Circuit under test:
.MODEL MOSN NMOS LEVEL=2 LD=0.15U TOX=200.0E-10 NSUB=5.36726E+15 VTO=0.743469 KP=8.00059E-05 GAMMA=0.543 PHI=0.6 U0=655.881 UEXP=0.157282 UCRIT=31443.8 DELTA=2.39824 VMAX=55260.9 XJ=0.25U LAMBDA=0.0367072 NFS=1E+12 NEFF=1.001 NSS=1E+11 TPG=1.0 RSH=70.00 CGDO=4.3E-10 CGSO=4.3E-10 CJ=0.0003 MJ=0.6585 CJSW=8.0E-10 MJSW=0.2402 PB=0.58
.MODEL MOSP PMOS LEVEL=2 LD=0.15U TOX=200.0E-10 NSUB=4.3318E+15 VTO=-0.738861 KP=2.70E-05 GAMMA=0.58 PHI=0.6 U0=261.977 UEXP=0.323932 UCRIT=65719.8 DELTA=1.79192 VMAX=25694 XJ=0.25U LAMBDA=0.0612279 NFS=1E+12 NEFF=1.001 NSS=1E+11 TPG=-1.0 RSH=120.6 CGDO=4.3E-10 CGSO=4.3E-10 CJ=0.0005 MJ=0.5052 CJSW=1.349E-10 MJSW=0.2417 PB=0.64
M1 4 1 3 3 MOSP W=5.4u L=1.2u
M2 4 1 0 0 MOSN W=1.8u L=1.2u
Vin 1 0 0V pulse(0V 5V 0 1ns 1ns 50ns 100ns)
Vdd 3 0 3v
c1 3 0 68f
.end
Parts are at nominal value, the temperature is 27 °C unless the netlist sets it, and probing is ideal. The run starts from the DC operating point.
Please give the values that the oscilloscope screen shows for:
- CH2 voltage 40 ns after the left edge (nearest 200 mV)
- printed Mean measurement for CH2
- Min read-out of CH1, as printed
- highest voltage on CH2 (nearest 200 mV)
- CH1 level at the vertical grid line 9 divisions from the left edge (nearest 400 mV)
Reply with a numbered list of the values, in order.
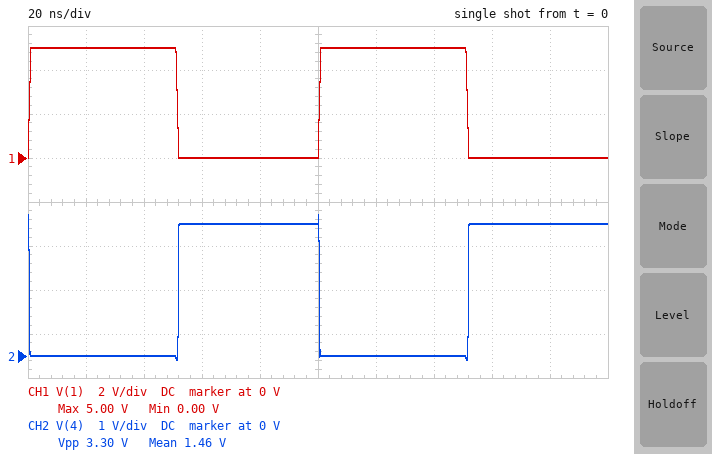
1. 0 V
2. 1.46 V
3. 0.00 V
4. 3.2 V
5. 0 V
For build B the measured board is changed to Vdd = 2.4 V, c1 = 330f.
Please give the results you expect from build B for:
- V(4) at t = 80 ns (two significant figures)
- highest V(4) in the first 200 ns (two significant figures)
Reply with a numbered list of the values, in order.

1. 2.4 V
2. 2.7 V
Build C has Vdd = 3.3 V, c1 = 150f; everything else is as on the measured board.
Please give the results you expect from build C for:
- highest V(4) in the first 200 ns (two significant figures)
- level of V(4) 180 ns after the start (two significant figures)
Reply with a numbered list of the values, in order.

1. 3.5 V
2. 3.3 V
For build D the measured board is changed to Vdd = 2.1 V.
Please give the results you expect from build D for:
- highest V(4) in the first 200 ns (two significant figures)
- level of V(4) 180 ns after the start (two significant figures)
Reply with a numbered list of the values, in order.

1. 2.4 V
2. 2.1 V
